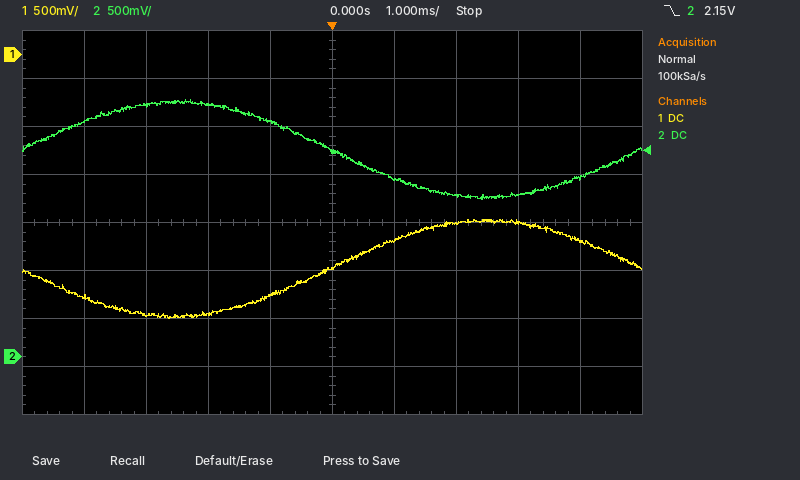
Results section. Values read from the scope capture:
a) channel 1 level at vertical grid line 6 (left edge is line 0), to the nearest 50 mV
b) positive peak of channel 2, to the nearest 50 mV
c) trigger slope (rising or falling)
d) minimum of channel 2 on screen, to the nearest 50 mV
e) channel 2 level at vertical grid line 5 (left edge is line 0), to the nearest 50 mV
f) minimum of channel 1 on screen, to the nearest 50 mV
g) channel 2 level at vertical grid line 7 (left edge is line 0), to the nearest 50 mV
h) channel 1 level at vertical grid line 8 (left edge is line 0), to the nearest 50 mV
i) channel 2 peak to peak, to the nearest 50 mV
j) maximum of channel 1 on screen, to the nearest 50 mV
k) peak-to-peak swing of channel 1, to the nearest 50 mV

-1.95 V
2.70 V
falling
1.65 V
2.15 V
-2.75 V
1.70 V
-1.75 V
1.05 V
-1.70 V
1.05 V
